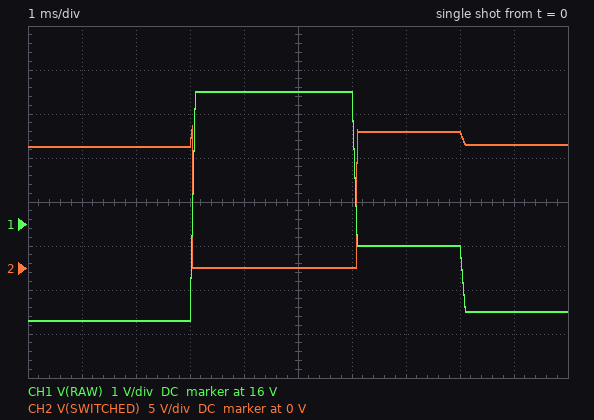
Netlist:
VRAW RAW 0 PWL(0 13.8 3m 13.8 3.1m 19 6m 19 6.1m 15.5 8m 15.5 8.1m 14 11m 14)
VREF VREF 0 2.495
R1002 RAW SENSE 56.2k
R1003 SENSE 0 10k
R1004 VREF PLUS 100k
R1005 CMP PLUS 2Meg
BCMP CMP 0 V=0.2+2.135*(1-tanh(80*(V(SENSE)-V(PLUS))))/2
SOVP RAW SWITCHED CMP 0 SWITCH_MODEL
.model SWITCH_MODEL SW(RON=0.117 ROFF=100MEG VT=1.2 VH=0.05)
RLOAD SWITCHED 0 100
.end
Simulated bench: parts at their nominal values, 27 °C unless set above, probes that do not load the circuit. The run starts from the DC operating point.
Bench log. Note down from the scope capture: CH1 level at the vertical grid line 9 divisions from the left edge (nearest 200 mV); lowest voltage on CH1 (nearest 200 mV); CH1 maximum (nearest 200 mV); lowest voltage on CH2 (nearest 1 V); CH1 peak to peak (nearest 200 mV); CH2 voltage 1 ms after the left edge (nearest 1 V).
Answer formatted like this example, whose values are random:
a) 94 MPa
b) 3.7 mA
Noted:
a) 14.0 V
b) 13.8 V
c) 19.0 V
d) 0 V
e) 5.2 V
f) 14 V
